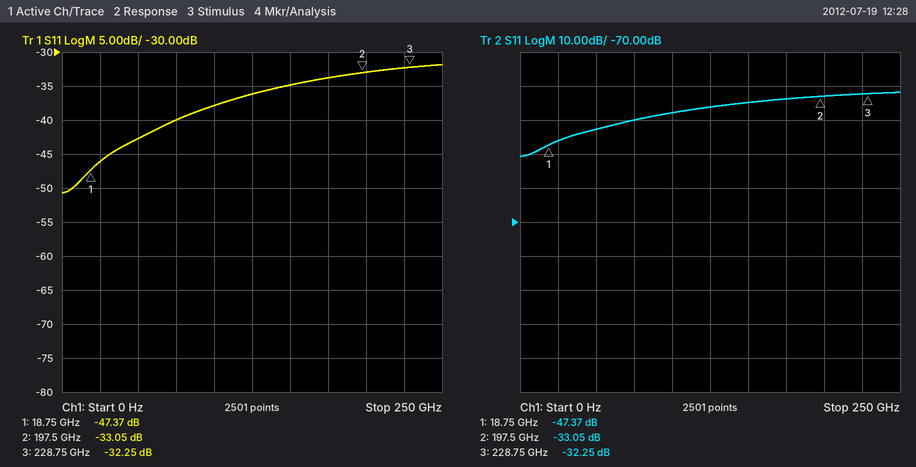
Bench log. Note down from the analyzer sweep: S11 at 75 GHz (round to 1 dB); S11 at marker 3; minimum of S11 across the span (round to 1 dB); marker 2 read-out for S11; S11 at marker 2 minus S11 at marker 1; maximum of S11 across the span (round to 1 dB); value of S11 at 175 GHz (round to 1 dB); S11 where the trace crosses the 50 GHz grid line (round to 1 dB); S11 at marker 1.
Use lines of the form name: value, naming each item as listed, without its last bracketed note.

S11 at 75 GHz: -40 dB
S11 at marker 3: -32.25 dB
minimum of S11 across the span: -51 dB
marker 2 read-out for S11: -33.05 dB
S11 at marker 2 minus S11 at marker 1: 14.32 dB
maximum of S11 across the span: -32 dB
value of S11 at 175 GHz: -34 dB
S11 where the trace crosses the 50 GHz grid line: -43 dB
S11 at marker 1: -47.37 dB
